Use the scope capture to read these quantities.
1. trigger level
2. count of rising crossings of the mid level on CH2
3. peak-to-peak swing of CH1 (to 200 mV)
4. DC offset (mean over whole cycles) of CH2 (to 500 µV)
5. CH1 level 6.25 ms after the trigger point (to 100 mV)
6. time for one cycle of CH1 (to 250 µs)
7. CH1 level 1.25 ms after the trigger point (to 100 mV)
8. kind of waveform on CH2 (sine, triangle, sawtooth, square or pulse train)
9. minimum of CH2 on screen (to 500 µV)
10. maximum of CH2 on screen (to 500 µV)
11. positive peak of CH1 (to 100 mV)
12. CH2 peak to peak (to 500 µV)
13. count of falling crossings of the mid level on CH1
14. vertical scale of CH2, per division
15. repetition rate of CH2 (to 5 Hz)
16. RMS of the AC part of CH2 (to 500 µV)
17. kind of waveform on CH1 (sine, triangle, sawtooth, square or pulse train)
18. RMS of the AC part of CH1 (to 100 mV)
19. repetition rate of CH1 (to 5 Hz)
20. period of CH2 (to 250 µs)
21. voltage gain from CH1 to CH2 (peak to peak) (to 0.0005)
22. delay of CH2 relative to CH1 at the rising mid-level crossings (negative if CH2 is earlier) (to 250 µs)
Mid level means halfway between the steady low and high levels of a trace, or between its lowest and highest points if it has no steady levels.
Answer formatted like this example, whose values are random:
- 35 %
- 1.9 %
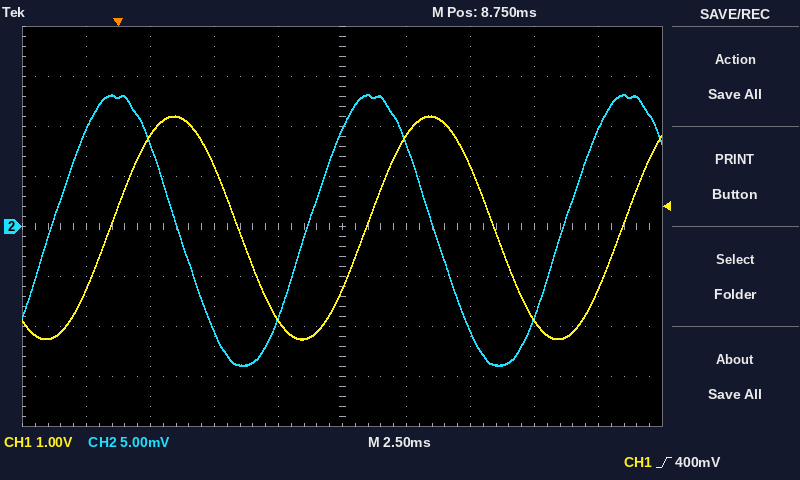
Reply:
- 400 mV
- 3
- 4.4 V
- -500 µV
- -1.9 V
- 10.00 ms
- 1.8 V
- sine
- -14.0 mV
- 13.0 mV
- 2.2 V
- 27.0 mV
- 2
- 5 mV
- 100 Hz
- 9.5 mV
- sine
- 1.6 V
- 100 Hz
- 10.00 ms
- 0.0060
- -2.25 ms
